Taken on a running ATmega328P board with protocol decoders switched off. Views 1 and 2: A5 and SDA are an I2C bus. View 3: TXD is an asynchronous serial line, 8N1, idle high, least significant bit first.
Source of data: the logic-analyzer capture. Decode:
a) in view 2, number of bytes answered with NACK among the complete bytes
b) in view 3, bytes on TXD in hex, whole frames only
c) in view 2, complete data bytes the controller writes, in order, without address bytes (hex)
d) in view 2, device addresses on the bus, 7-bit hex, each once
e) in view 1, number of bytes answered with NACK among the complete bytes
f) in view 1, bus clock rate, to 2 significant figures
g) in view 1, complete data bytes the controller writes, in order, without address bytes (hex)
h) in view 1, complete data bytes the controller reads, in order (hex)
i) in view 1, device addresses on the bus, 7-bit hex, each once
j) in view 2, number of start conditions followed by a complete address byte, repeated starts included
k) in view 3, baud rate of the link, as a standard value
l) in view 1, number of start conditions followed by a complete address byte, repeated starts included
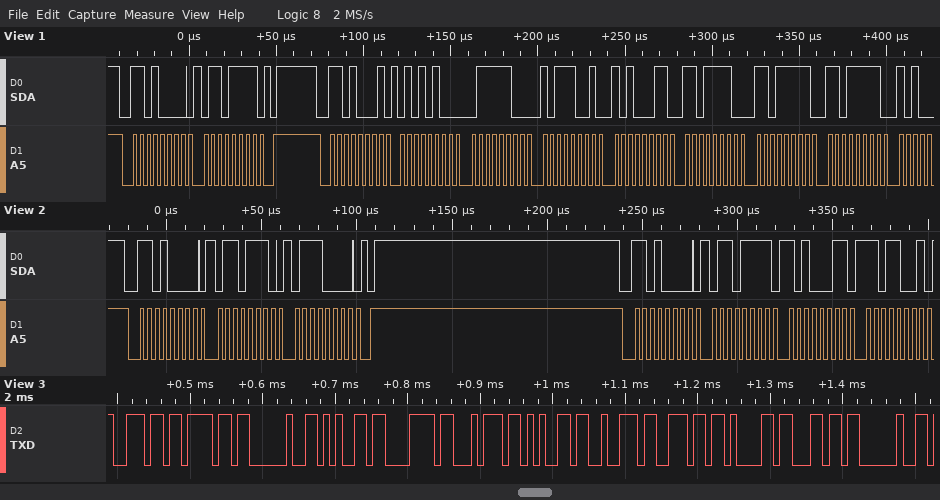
0
6E 6F 20 65 78 74 65 72 6E 61 6C 20
6E 70 6F A3 D9
0x68
0
250 kHz
6F
54 7C B9 A3 DE DF DF
0x68
2
115200 baud
2
